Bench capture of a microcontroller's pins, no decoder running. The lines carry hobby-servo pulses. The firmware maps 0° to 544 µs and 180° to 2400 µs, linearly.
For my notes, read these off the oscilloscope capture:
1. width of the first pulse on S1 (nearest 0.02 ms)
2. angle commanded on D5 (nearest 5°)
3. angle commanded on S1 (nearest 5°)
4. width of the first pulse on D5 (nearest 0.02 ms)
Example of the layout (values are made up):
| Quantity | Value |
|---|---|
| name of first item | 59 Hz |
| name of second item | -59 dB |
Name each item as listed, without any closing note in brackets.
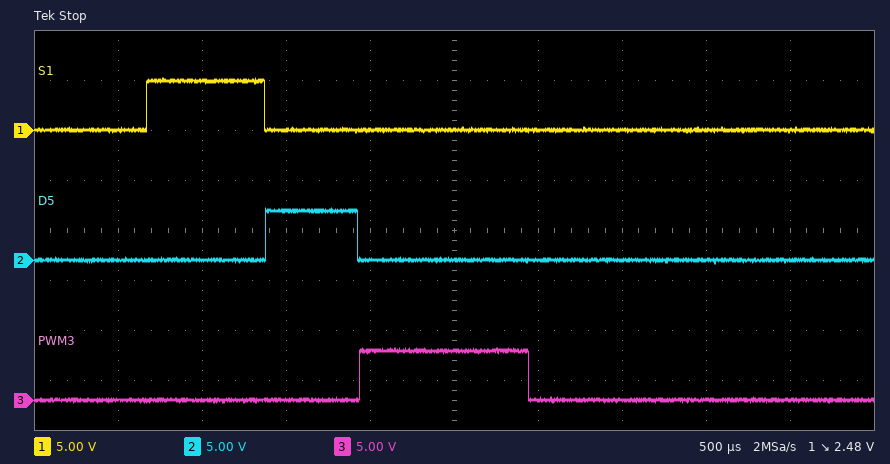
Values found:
| Quantity | Value |
|---|---|
| width of the first pulse on S1 | 0.70 ms |
| angle commanded on D5 | 0° |
| angle commanded on S1 | 15° |
| width of the first pulse on D5 | 0.54 ms |
